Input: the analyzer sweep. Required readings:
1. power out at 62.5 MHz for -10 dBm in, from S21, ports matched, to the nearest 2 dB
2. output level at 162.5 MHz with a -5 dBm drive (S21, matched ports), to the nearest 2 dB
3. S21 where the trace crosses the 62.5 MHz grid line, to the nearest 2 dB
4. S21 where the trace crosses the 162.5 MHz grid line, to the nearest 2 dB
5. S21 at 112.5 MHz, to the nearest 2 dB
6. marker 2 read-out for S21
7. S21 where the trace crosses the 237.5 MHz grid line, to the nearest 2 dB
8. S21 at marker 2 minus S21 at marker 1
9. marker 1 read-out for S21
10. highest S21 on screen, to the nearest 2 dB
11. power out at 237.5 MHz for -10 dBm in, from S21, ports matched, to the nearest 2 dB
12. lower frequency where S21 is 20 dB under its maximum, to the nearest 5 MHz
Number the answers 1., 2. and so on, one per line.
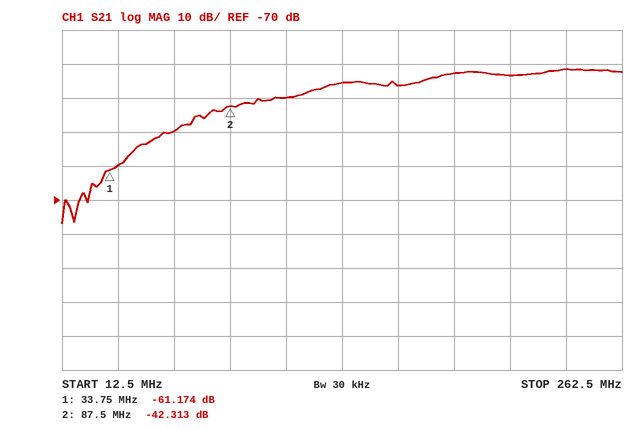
1. -60 dBm
2. -42 dBm
3. -50 dB
4. -36 dB
5. -40 dB
6. -42.313 dB
7. -32 dB
8. 18.861 dB
9. -61.174 dB
10. -32 dB
11. -42 dBm
12. 55 MHz
